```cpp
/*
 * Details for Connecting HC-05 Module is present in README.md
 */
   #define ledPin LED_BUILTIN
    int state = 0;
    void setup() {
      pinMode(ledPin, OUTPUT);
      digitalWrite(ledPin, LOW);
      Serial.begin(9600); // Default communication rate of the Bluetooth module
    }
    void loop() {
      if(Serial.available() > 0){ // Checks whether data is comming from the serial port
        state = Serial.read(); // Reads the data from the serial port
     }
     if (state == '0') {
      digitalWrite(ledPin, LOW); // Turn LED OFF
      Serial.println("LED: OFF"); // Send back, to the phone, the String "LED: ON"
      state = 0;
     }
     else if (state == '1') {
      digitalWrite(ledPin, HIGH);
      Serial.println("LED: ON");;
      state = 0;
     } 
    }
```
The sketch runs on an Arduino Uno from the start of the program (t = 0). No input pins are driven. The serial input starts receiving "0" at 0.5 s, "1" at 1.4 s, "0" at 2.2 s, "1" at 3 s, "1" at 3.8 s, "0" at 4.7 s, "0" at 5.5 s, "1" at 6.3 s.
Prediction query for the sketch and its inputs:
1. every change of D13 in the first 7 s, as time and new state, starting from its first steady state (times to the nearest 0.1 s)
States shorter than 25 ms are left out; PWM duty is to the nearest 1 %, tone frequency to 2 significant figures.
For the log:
0 s low; 1.4 s high; 2.2 s low; 3 s high; 4.7 s low; 6.3 s high
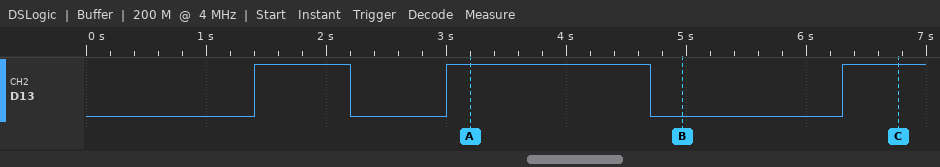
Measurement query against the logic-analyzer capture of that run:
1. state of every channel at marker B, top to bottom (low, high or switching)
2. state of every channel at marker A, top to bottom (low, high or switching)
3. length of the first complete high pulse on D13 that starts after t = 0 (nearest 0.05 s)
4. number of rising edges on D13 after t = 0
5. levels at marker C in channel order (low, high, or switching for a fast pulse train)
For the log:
D13 low
D13 high
0.80 s
3
D13 high
